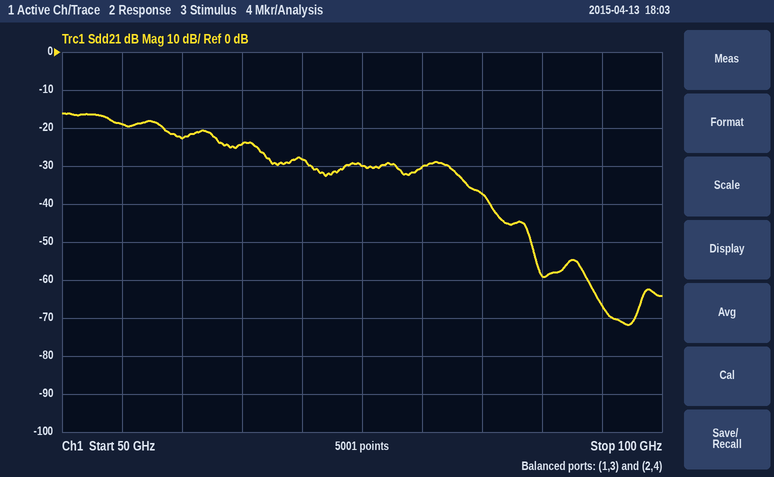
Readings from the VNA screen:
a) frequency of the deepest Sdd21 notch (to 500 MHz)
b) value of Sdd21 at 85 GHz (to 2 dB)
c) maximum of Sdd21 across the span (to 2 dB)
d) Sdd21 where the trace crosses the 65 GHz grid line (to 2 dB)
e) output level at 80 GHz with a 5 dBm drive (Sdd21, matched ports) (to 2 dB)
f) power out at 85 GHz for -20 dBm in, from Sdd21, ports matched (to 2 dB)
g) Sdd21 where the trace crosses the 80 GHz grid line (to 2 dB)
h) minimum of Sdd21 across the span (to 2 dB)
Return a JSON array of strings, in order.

["97.0 GHz", "-38 dB", "-16 dB", "-24 dB", "-26 dBm", "-58 dBm", "-30 dB", "-72 dB"]
